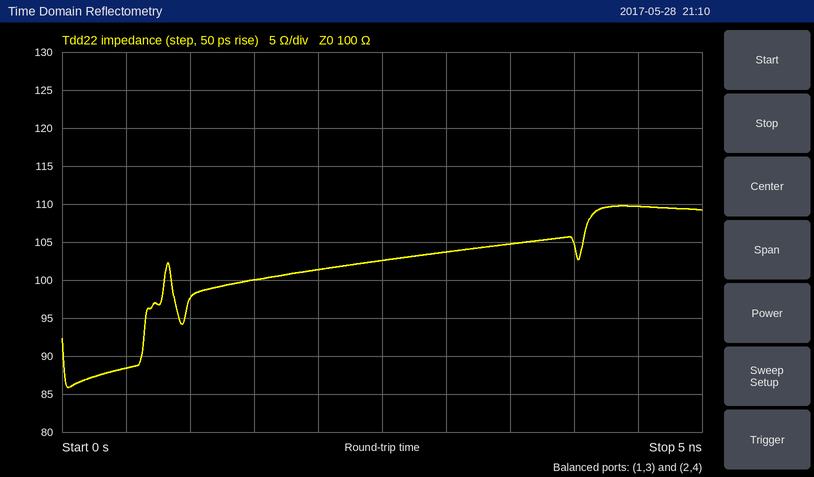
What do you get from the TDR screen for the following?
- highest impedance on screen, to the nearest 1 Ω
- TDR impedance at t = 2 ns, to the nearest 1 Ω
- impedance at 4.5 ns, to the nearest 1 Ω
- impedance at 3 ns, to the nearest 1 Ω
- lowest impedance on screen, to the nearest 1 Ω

110 Ω
101 Ω
110 Ω
104 Ω
86 Ω
